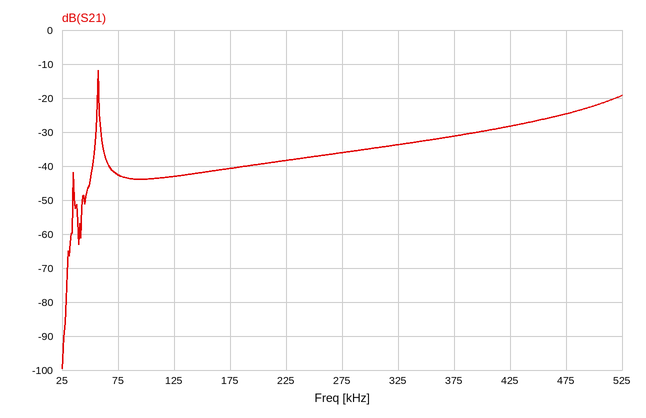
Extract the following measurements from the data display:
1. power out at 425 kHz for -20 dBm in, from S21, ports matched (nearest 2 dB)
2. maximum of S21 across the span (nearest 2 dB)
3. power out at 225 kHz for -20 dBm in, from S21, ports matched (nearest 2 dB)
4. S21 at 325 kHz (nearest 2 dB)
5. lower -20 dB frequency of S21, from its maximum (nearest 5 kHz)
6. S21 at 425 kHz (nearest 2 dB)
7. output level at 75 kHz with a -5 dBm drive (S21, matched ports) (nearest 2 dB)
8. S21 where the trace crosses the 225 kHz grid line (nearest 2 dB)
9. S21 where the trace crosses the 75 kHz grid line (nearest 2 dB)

-48 dBm
-12 dB
-58 dBm
-34 dB
55 kHz
-28 dB
-48 dBm
-38 dB
-42 dB
